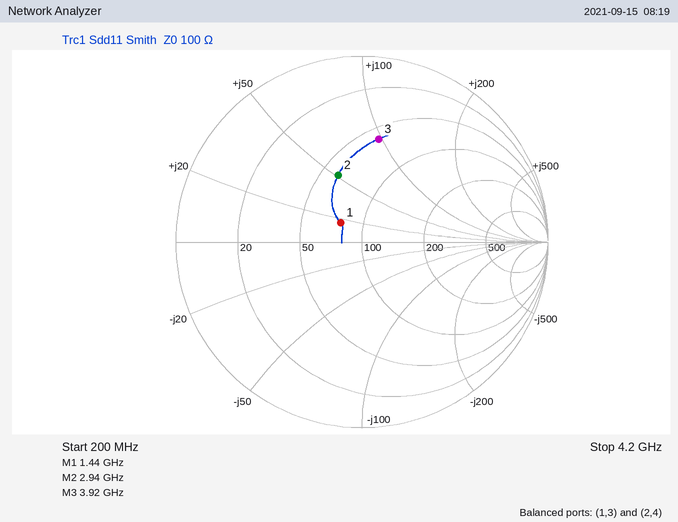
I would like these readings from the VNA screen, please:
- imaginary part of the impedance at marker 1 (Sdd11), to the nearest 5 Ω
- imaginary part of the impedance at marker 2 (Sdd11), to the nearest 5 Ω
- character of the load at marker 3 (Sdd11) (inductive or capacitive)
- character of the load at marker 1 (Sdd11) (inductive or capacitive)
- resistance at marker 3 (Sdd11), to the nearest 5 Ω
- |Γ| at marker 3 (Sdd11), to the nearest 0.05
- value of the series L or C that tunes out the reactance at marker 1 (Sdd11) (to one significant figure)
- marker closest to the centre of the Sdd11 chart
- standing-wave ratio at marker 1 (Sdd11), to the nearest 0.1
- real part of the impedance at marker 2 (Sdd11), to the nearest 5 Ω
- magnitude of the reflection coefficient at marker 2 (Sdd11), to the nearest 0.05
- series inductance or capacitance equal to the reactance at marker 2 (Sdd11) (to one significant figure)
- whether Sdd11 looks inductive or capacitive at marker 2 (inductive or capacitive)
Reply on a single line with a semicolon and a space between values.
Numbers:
+15 Ω; +50 Ω; inductive; inductive; 60 Ω; 0.55; 7 pF; marker 1; 1.4; 60 Ω; 0.40; 3 nH; inductive
